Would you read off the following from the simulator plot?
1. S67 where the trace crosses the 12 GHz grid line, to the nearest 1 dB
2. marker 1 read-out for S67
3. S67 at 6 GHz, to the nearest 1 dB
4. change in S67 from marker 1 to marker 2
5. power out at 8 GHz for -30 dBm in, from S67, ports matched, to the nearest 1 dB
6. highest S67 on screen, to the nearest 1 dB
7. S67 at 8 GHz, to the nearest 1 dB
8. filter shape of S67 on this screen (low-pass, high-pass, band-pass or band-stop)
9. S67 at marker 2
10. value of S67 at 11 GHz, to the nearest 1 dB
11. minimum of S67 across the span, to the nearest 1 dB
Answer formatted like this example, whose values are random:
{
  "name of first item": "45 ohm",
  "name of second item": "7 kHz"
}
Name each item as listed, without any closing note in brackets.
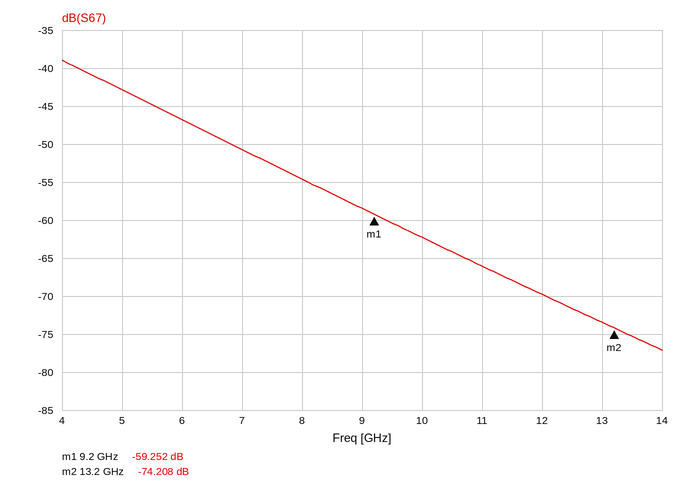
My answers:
{
  "S67 where the trace crosses the 12 GHz grid line, to the nearest 1 dB": "-70 dB",
  "marker 1 read-out for S67": "-59.252 dB",
  "S67 at 6 GHz, to the nearest 1 dB": "-47 dB",
  "change in S67 from marker 1 to marker 2": "-14.956 dB",
  "power out at 8 GHz for -30 dBm in, from S67, ports matched, to the nearest 1 dB": "-85 dBm",
  "highest S67 on screen, to the nearest 1 dB": "-39 dB",
  "S67 at 8 GHz, to the nearest 1 dB": "-55 dB",
  "filter shape of S67 on this screen": "low-pass",
  "S67 at marker 2": "-74.208 dB",
  "value of S67 at 11 GHz, to the nearest 1 dB": "-66 dB",
  "minimum of S67 across the span, to the nearest 1 dB": "-77 dB"
}
